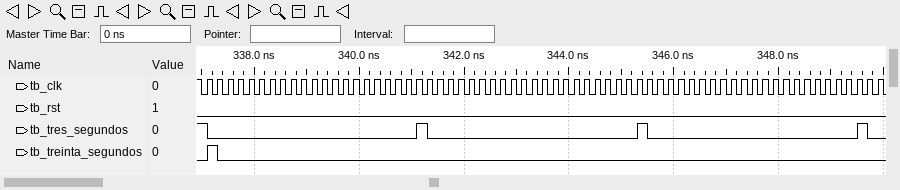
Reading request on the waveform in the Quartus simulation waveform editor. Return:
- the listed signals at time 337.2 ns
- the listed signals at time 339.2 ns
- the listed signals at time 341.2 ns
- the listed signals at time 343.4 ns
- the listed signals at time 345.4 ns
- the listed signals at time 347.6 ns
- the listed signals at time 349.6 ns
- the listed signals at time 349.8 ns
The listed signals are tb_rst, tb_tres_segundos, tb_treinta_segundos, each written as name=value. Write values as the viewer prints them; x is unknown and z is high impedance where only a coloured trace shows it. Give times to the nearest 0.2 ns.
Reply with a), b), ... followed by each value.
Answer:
a) tb_rst=0, tb_tres_segundos=0, tb_treinta_segundos=1
b) tb_rst=0, tb_tres_segundos=0, tb_treinta_segundos=0
c) tb_rst=0, tb_tres_segundos=1, tb_treinta_segundos=0
d) tb_rst=0, tb_tres_segundos=0, tb_treinta_segundos=0
e) tb_rst=0, tb_tres_segundos=1, tb_treinta_segundos=0
f) tb_rst=0, tb_tres_segundos=0, tb_treinta_segundos=0
g) tb_rst=0, tb_tres_segundos=1, tb_treinta_segundos=0
h) tb_rst=0, tb_tres_segundos=0, tb_treinta_segundos=0
